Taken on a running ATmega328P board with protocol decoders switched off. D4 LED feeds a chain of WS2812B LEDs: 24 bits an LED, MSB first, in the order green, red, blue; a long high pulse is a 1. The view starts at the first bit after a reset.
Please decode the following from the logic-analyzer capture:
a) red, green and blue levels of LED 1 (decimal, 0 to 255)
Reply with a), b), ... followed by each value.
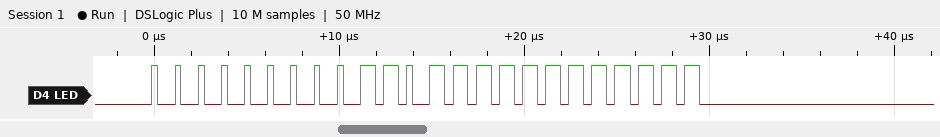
a) 111, 0, 255
